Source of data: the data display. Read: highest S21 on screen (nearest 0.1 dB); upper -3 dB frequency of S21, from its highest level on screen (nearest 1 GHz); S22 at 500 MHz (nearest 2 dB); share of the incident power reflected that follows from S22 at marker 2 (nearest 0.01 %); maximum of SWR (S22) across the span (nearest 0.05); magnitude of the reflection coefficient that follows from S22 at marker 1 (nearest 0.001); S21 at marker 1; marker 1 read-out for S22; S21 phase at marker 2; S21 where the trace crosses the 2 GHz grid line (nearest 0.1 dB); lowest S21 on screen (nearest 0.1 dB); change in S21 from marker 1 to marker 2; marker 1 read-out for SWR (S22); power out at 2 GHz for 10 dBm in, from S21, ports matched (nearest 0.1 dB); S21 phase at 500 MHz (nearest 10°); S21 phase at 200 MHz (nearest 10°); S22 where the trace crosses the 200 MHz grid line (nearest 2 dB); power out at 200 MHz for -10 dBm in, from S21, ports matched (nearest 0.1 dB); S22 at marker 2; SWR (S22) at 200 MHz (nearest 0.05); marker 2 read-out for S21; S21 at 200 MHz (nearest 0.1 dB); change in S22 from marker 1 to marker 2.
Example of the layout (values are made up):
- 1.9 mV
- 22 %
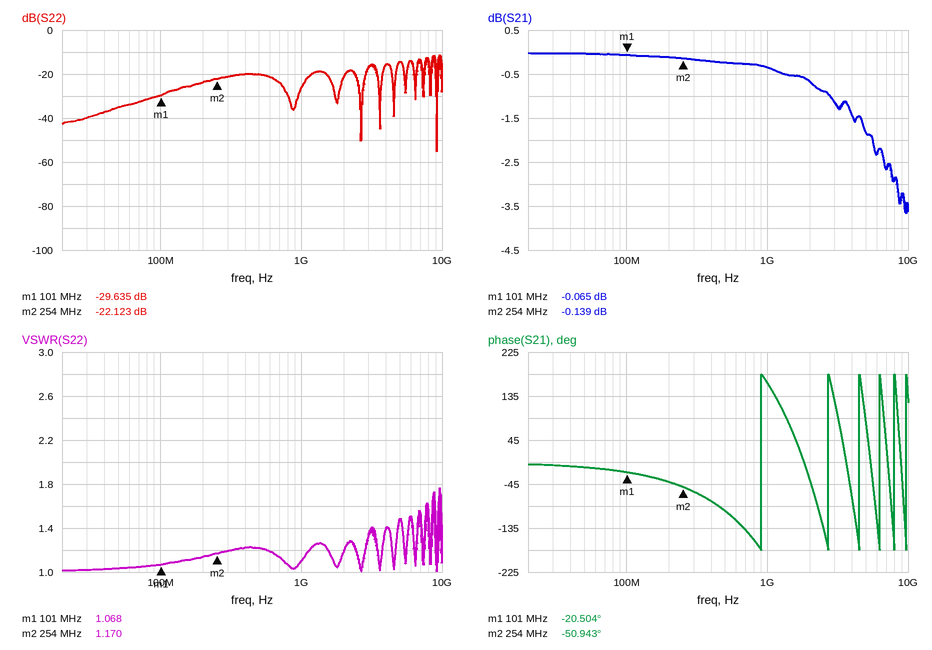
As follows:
- 0.0 dB
- 8 GHz
- -20 dB
- 0.61 %
- 1.75
- 0.033
- -0.065 dB
- -29.635 dB
- -50.943°
- -0.7 dB
- -3.7 dB
- -0.074 dB
- 1.068
- 9.3 dBm
- -100°
- -40°
- -24 dB
- -10.1 dBm
- -22.123 dB
- 1.15
- -0.139 dB
- -0.1 dB
- 7.512 dB
